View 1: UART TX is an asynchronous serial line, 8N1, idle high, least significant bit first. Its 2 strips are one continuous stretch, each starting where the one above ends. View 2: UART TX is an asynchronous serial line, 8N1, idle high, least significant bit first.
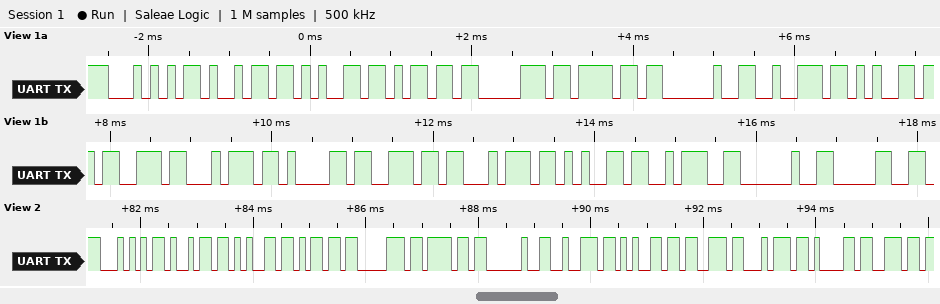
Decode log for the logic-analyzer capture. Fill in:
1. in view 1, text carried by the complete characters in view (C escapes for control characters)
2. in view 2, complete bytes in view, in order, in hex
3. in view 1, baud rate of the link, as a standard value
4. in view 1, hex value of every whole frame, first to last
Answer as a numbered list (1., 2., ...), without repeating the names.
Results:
1. "Tiempo restante: 0"
2. 0x54 0x69 0x65 0x6D 0x70 0x6F 0x20 0x72 0x65 0x73 0x74 0x61 0x6E
3. 9600 baud
4. 54 69 65 6D 70 6F 20 72 65 73 74 61 6E 74 65 3A 20 30
